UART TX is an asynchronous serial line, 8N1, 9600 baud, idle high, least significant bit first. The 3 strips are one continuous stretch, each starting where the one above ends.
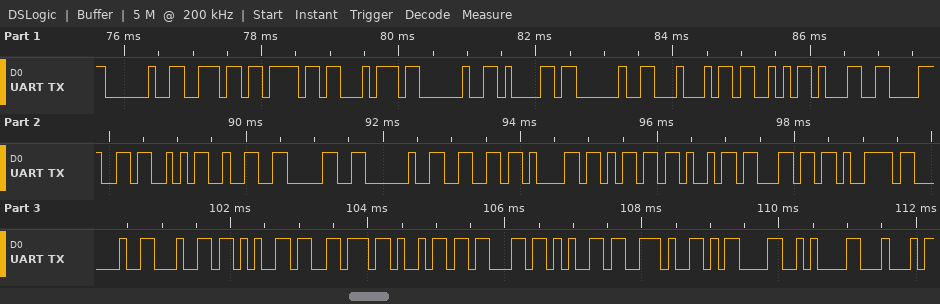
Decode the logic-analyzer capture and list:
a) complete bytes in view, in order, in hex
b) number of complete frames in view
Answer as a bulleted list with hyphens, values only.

- 20 6E 6F 74 20 61 20 44 53 31 38 53 32 30 20 66 61 6D 69 6C 79 20 64 65 76 69 63 65 2E 0D 0A 44
- 32
